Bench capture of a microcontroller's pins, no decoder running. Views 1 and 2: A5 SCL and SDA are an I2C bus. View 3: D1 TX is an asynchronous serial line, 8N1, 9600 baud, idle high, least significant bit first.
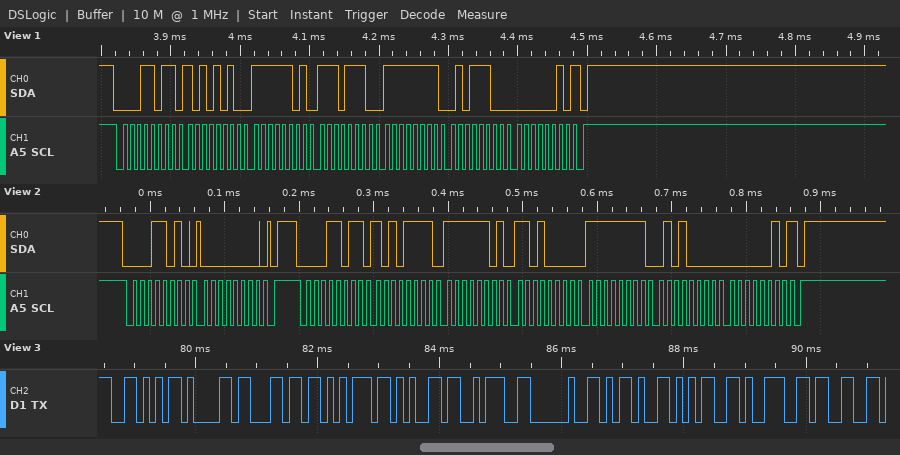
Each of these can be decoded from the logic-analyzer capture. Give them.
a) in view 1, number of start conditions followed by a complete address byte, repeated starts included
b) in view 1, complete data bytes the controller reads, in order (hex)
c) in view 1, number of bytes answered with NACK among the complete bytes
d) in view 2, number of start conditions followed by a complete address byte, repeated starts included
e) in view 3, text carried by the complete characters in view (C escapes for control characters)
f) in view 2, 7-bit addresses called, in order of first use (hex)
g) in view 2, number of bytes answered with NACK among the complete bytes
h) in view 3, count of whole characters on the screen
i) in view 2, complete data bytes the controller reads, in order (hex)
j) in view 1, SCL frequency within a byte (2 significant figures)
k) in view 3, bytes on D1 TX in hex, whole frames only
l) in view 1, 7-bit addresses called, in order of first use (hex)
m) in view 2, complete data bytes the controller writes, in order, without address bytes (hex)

1
AA FD EE FF 5C 02
1
2
"Value: -593"
0x0D
1
11
AF FD D0 FF 50 02
100 kHz
56 61 6C 75 65 3A 20 2D 35 39 33
0x0D
00
